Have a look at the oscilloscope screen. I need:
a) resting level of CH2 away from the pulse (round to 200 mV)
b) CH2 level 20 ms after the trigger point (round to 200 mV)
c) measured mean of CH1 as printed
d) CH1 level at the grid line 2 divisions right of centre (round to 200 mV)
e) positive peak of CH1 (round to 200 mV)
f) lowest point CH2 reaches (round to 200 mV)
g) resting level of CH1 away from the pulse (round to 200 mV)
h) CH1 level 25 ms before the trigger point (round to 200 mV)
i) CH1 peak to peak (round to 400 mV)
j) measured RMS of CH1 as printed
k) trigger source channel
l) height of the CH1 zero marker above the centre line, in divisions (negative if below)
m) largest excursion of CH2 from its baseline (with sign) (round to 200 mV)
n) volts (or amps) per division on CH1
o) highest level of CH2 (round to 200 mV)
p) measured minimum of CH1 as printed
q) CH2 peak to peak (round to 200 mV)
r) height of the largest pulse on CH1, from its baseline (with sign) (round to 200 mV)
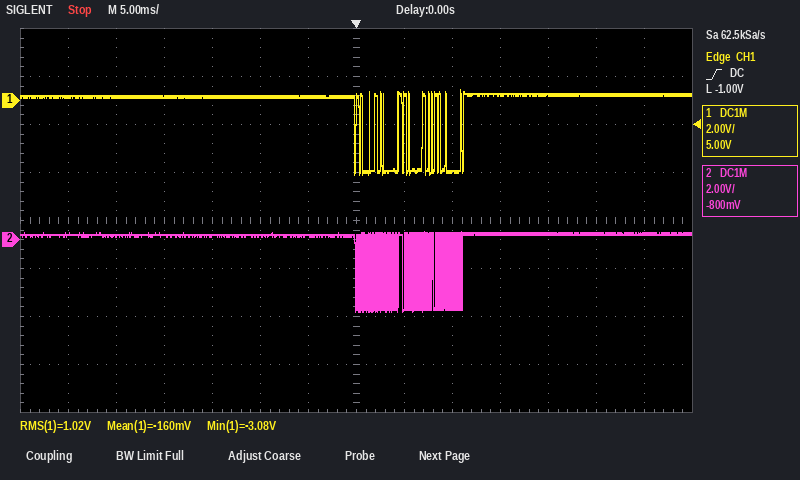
200 mV
200 mV
-160 mV
-3.0 V
400 mV
-3.0 V
200 mV
200 mV
3.6 V
1.02 V
CH1
+2.5 div
-3.2 V
2 V
400 mV
-3.08 V
3.4 V
-3.2 V
